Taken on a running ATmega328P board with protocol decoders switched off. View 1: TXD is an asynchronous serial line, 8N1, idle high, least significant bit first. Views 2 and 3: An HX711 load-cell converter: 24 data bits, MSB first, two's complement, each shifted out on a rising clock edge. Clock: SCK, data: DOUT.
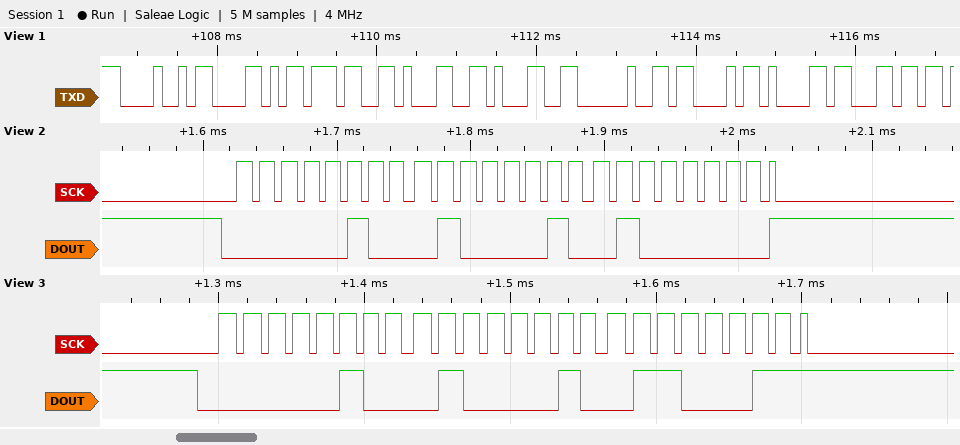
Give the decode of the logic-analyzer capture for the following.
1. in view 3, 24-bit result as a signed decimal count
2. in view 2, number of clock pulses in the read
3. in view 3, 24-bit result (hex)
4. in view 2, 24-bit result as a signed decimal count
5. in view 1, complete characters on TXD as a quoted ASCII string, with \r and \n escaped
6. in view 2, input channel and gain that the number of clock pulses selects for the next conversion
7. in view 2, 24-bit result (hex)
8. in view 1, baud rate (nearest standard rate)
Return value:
279139
25
0x044263
279104
"HX711 Cal"
channel A, gain 128
0x044240
9600 baud
